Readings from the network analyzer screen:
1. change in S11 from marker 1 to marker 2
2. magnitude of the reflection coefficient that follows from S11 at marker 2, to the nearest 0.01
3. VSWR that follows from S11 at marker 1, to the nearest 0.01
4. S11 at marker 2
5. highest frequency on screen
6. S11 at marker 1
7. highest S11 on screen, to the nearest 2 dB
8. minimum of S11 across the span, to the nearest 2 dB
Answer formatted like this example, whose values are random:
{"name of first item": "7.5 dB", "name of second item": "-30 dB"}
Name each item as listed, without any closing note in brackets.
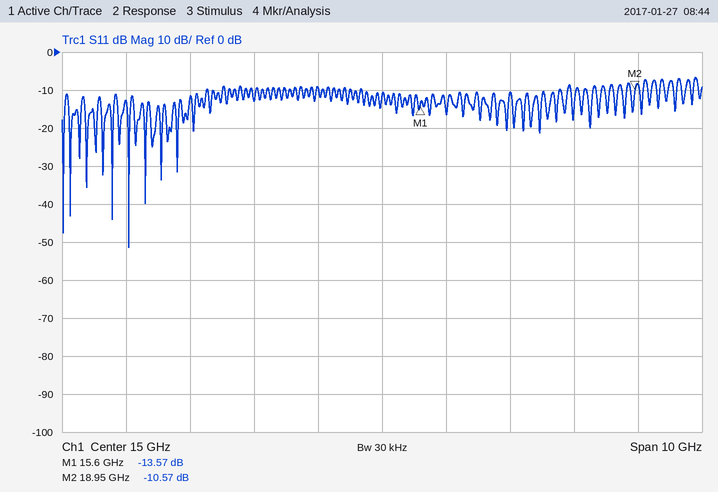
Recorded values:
{"change in S11 from marker 1 to marker 2": "3.00 dB", "magnitude of the reflection coefficient that follows from S11 at marker 2, to the nearest 0.01": "0.30", "VSWR that follows from S11 at marker 1, to the nearest 0.01": "1.53", "S11 at marker 2": "-10.57 dB", "highest frequency on screen": "20 GHz", "S11 at marker 1": "-13.57 dB", "highest S11 on screen, to the nearest 2 dB": "-6 dB", "minimum of S11 across the span, to the nearest 2 dB": "-52 dB"}
